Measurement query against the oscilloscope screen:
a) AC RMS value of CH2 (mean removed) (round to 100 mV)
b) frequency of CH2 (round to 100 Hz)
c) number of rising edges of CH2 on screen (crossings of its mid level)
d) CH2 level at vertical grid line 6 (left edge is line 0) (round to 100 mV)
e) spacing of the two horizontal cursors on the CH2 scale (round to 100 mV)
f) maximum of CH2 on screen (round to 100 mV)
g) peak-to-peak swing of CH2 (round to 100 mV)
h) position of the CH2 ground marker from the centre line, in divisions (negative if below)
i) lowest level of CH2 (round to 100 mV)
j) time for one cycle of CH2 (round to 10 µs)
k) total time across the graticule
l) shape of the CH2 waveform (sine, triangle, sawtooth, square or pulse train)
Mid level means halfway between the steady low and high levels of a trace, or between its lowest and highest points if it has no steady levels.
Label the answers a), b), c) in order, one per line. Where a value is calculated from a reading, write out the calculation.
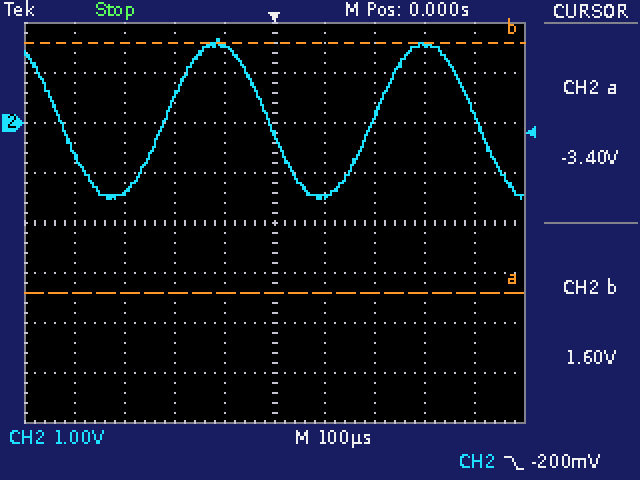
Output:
a) 3.2 V / (2√2) ≈ 1.1 V
b) 1 / 420 µs ≈ 2.4 kHz
c) 2
d) -1.5 V
e) 5.0 V
f) 1.7 V
g) 1.7 V − (-1.5 V) = 3.2 V
h) +2.0 div
i) -1.5 V
j) 420 µs
k) 1 ms
l) sine
